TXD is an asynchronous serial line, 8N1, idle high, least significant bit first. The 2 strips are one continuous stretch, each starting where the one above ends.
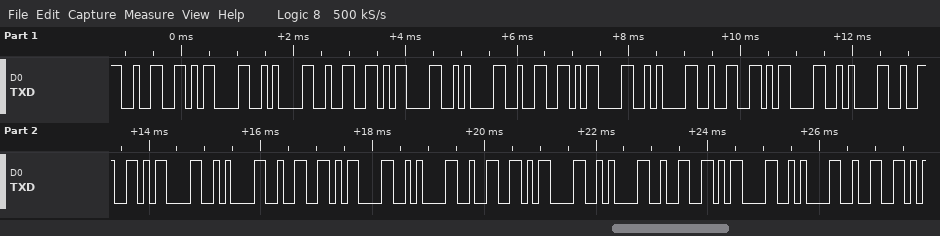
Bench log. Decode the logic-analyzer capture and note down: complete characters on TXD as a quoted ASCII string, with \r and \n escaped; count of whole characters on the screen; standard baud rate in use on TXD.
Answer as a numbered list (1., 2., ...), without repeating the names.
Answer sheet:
1. "2\r\n2\r\n2\r\n2\r\n2\r\n2\r\n2\r\n2\r\n2"
2. 25
3. 9600 baud
